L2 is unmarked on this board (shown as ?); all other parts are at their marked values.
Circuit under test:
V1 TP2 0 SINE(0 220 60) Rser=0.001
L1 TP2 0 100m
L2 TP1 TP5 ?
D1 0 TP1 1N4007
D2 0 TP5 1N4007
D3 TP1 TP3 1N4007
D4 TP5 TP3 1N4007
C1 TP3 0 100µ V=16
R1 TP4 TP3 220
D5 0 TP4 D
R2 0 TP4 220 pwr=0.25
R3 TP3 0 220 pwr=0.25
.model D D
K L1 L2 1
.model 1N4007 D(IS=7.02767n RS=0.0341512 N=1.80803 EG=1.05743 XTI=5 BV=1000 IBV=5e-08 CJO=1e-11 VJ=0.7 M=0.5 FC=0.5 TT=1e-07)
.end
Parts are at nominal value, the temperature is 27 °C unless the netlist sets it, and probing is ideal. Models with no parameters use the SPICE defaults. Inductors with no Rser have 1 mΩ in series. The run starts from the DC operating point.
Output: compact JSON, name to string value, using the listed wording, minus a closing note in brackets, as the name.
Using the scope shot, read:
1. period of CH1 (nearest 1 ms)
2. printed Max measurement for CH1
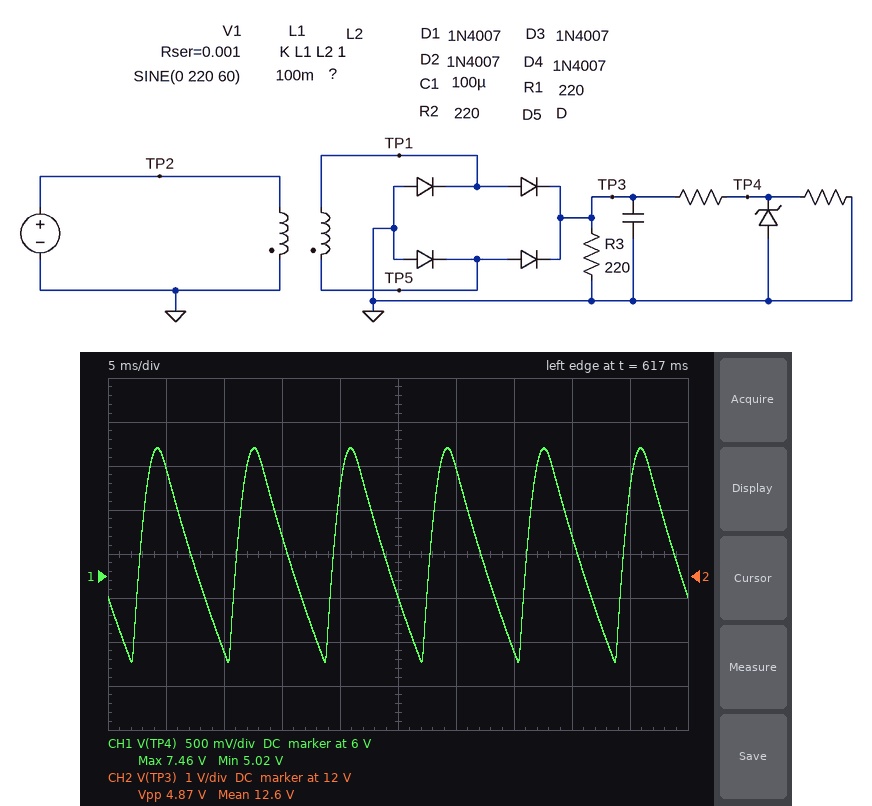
{"period of CH1": "8 ms", "printed Max measurement for CH1": "7.46 V"}
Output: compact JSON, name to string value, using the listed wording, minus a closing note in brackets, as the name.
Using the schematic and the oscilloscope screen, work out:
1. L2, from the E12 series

{"L2, from the E12 series": "560 µH"}
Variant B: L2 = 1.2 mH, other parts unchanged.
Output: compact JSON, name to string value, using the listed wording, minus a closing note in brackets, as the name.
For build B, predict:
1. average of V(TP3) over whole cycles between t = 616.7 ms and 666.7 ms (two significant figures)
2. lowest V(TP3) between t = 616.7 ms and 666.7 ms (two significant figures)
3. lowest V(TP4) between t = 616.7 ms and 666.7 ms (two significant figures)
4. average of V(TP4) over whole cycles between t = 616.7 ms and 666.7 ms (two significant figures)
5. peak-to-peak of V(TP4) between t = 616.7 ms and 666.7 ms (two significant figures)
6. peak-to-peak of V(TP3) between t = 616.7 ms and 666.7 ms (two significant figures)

{"average of V(TP3) over whole cycles between t = 616.7 ms and 666.7 ms": "19 V", "lowest V(TP3) between t = 616.7 ms and 666.7 ms": "15 V", "lowest V(TP4) between t = 616.7 ms and 666.7 ms": "7.6 V", "average of V(TP4) over whole cycles between t = 616.7 ms and 666.7 ms": "9.5 V", "peak-to-peak of V(TP4) between t = 616.7 ms and 666.7 ms": "3.7 V", "peak-to-peak of V(TP3) between t = 616.7 ms and 666.7 ms": "7.4 V"}
